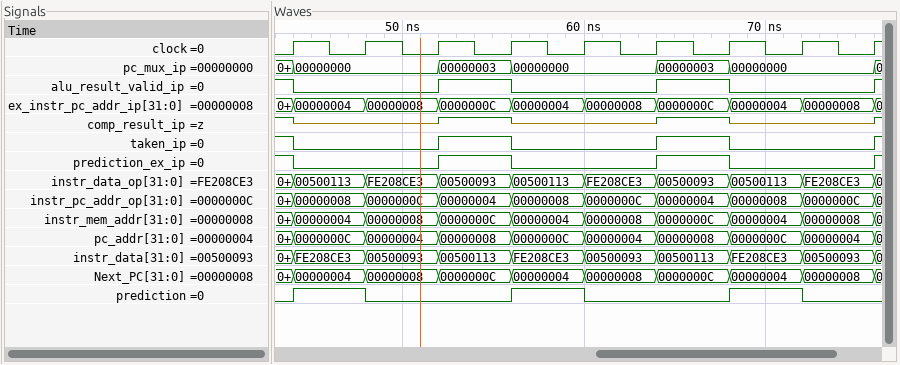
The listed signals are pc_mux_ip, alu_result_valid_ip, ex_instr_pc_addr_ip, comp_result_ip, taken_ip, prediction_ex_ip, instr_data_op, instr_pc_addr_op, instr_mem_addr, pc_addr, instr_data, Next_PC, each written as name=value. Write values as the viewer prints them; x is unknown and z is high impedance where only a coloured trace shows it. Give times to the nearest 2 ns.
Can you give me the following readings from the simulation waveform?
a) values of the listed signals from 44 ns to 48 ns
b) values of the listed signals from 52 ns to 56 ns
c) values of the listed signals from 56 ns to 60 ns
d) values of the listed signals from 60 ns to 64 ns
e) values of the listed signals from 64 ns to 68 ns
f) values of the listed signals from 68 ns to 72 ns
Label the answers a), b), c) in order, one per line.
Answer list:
a) pc_mux_ip=00000000, alu_result_valid_ip=0, ex_instr_pc_addr_ip=00000004, comp_result_ip=z, taken_ip=0, prediction_ex_ip=0, instr_data_op=00500113, instr_pc_addr_op=00000008, instr_mem_addr=00000004, pc_addr=0000000C, instr_data=FE208CE3, Next_PC=00000004
b) pc_mux_ip=00000003, alu_result_valid_ip=1, ex_instr_pc_addr_ip=0000000C, comp_result_ip=1, taken_ip=1, prediction_ex_ip=1, instr_data_op=00500093, instr_pc_addr_op=00000004, instr_mem_addr=0000000C, pc_addr=00000008, instr_data=00500113, Next_PC=0000000C
c) pc_mux_ip=00000000, alu_result_valid_ip=0, ex_instr_pc_addr_ip=00000004, comp_result_ip=z, taken_ip=0, prediction_ex_ip=0, instr_data_op=00500113, instr_pc_addr_op=00000008, instr_mem_addr=00000004, pc_addr=0000000C, instr_data=FE208CE3, Next_PC=00000004
d) pc_mux_ip=00000000, alu_result_valid_ip=0, ex_instr_pc_addr_ip=00000008, comp_result_ip=z, taken_ip=0, prediction_ex_ip=0, instr_data_op=FE208CE3, instr_pc_addr_op=0000000C, instr_mem_addr=00000008, pc_addr=00000004, instr_data=00500093, Next_PC=00000008
e) pc_mux_ip=00000003, alu_result_valid_ip=1, ex_instr_pc_addr_ip=0000000C, comp_result_ip=1, taken_ip=1, prediction_ex_ip=1, instr_data_op=00500093, instr_pc_addr_op=00000004, instr_mem_addr=0000000C, pc_addr=00000008, instr_data=00500113, Next_PC=0000000C
f) pc_mux_ip=00000000, alu_result_valid_ip=0, ex_instr_pc_addr_ip=00000004, comp_result_ip=z, taken_ip=0, prediction_ex_ip=0, instr_data_op=00500113, instr_pc_addr_op=00000008, instr_mem_addr=00000004, pc_addr=0000000C, instr_data=FE208CE3, Next_PC=00000004
